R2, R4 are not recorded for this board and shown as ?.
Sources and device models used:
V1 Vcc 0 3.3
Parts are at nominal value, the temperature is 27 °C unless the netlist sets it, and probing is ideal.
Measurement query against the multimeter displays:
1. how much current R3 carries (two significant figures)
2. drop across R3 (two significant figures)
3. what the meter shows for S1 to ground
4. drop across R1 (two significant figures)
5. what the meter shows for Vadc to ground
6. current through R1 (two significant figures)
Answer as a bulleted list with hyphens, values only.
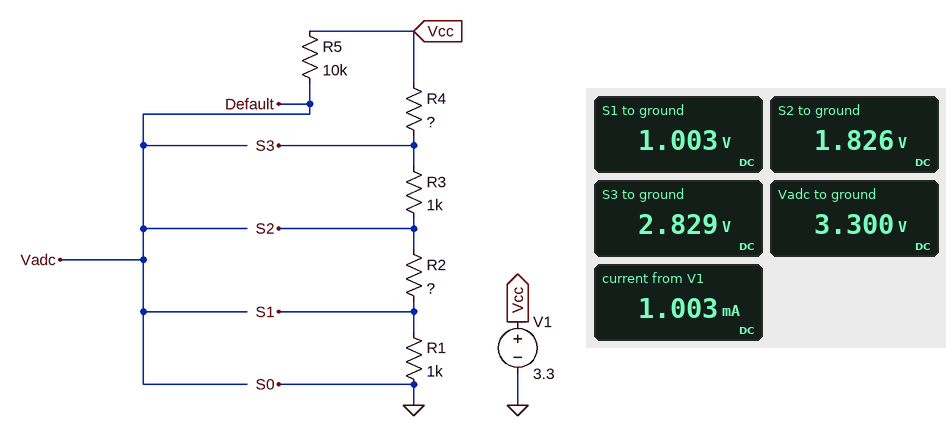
- 1.0 mA
- 1.0 V
- 1.003 V
- 1.0 V
- 3.300 V
- 1.0 mA
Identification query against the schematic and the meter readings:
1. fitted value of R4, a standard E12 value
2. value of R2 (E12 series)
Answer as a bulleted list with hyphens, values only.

- 470 Ω
- 820 Ω
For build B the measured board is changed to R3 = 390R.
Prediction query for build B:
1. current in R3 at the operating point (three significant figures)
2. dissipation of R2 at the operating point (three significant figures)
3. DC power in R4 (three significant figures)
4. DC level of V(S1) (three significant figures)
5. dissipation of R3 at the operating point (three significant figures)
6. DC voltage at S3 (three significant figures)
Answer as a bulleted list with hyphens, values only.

- 1.23 mA
- 1.24 mW
- 713 µW
- 1.23 V
- 591 µW
- 2.72 V
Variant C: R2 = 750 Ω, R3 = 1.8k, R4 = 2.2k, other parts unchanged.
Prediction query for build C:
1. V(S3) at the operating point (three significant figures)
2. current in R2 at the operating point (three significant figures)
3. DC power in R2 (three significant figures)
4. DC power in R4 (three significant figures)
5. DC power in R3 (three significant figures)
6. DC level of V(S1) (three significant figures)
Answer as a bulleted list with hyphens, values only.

- 2.04 V
- 574 µA
- 247 µW
- 725 µW
- 593 µW
- 574 mV
